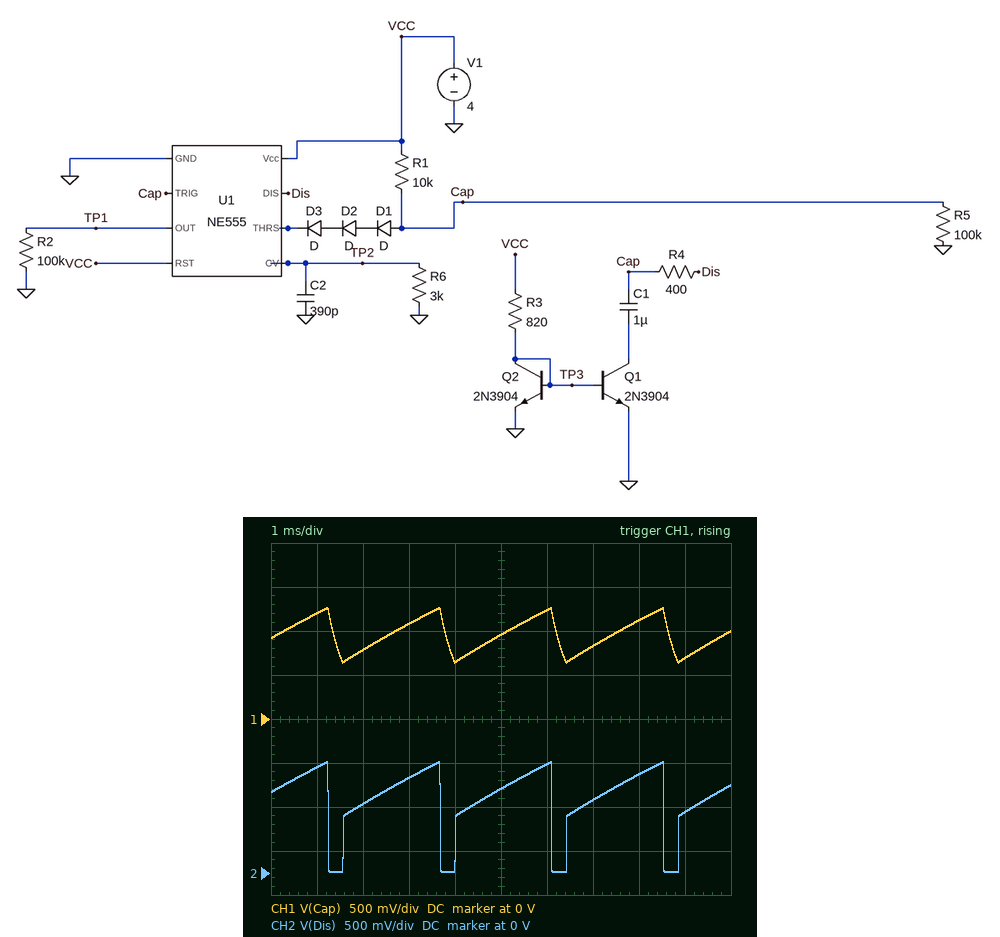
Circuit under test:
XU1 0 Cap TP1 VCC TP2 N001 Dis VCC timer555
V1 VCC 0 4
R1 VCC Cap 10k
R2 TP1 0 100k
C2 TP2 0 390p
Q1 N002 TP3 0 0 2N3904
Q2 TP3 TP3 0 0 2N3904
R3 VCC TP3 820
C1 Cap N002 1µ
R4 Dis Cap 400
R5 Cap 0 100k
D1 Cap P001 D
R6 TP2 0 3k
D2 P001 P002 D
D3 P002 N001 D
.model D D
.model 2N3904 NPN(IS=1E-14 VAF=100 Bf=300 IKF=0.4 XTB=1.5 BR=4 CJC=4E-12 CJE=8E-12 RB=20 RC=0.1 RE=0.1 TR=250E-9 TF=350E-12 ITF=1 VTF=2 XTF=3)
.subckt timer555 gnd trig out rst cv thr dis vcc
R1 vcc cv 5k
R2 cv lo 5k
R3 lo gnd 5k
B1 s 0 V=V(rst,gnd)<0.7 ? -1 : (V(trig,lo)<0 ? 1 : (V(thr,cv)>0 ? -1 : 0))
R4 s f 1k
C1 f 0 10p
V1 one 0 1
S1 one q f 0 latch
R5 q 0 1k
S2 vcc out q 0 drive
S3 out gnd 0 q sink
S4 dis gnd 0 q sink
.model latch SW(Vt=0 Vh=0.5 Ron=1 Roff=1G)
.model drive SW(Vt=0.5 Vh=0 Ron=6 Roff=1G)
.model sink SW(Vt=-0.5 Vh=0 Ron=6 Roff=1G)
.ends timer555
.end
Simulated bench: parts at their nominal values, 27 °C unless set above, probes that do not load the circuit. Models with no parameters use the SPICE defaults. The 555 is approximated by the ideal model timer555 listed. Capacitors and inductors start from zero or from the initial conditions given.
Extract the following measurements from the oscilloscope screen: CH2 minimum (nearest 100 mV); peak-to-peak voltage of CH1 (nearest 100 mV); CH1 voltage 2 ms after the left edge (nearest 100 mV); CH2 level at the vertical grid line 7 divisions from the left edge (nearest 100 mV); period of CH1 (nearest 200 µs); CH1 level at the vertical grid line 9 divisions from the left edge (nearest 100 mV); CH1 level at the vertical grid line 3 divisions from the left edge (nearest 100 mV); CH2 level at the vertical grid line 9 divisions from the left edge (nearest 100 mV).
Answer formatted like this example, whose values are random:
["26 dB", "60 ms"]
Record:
["0 V", "600 mV", "800 mV", "800 mV", "2.4 ms", "700 mV", "1.1 V", "700 mV"]
